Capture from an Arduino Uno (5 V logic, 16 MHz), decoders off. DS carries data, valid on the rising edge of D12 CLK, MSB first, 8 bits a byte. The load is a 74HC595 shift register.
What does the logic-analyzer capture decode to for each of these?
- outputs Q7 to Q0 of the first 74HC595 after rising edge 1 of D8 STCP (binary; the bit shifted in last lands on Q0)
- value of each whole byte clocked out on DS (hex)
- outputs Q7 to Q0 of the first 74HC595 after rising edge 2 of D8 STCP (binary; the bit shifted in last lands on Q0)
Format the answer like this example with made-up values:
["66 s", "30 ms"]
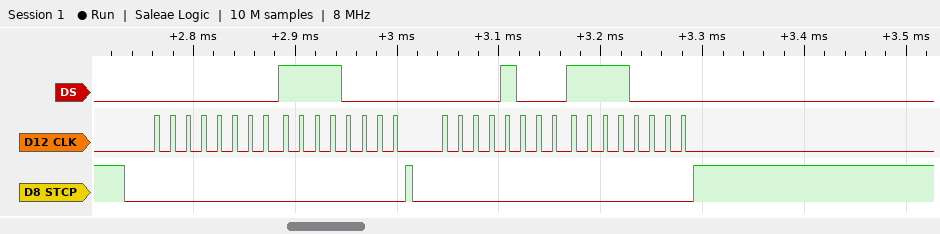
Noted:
["11110000", "00 F0 08 F0", "11110000"]
